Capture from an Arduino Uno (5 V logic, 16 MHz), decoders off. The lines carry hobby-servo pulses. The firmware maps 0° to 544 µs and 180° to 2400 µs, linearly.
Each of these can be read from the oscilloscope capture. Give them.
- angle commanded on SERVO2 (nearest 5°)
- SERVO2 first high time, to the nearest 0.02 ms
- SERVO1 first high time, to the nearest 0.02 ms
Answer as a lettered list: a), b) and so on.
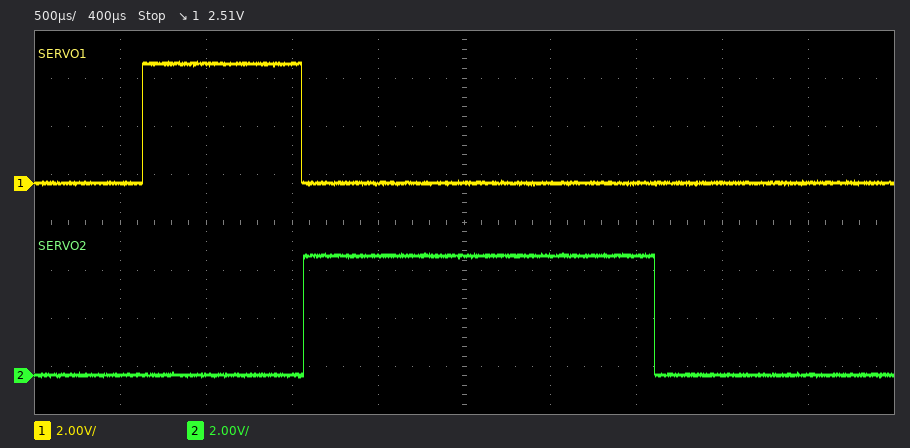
a) 145°
b) 2.04 ms
c) 0.92 ms
